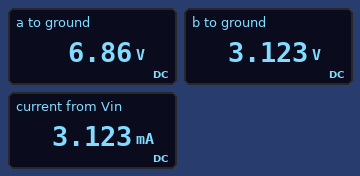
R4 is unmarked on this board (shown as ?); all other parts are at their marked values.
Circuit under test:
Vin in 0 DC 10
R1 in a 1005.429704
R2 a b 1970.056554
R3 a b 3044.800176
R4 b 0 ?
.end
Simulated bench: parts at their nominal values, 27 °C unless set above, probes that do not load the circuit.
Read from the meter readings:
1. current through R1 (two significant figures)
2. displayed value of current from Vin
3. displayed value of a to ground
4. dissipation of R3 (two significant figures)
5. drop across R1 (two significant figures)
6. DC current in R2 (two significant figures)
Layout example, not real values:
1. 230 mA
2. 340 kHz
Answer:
1. 3.1 mA
2. 3.123 mA
3. 6.86 V
4. 4.6 mW
5. 3.1 V
6. 1.9 mA
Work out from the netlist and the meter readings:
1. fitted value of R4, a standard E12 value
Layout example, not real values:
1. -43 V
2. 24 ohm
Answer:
1. 1 kΩ
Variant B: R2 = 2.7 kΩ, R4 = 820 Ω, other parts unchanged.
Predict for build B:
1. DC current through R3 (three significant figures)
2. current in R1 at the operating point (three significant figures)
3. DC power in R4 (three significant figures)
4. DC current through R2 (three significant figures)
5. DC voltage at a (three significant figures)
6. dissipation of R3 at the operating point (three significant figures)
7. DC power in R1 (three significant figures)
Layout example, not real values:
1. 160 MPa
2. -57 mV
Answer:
1. 1.44 mA
2. 3.07 mA
3. 7.73 mW
4. 1.63 mA
5. 6.91 V
6. 6.34 mW
7. 9.48 mW
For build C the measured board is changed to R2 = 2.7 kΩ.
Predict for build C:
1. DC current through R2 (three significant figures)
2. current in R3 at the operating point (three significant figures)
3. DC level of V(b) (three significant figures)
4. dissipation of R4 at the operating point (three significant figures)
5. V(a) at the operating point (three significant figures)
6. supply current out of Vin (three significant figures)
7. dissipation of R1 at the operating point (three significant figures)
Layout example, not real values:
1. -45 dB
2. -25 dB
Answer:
1. 1.54 mA
2. 1.37 mA
3. 2.91 V
4. 8.47 mW
5. 7.07 V
6. 2.91 mA
7. 8.51 mW
